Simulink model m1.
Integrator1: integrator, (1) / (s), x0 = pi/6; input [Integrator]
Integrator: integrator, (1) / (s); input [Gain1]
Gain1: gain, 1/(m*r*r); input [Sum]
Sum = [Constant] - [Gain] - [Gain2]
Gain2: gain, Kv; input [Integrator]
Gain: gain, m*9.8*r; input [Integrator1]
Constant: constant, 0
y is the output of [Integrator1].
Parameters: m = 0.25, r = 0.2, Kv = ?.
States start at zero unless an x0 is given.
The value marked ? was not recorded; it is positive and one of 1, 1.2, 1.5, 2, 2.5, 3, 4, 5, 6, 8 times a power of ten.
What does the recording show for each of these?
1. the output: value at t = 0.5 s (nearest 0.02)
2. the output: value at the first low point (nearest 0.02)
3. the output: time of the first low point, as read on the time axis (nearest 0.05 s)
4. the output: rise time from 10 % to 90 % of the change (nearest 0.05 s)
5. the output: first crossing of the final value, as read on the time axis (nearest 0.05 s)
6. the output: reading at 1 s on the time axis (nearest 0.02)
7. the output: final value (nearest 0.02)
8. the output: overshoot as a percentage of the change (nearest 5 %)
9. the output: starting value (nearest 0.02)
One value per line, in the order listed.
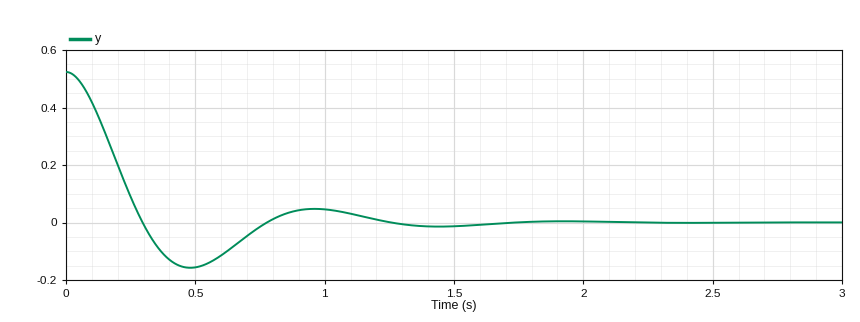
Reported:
-0.16
-0.16
0.50 s
0.20 s
0.30 s
0.04
0.00
30 %
0.52
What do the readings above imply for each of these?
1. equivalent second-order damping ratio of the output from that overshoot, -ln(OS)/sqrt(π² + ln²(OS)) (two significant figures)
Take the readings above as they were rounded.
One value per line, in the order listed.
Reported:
0.36
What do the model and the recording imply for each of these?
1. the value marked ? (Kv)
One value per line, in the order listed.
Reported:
0.05
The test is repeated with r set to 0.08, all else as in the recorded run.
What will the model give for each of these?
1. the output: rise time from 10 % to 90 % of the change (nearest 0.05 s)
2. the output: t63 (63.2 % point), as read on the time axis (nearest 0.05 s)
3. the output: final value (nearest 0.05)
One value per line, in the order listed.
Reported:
0.50 s
0.25 s
0.00
